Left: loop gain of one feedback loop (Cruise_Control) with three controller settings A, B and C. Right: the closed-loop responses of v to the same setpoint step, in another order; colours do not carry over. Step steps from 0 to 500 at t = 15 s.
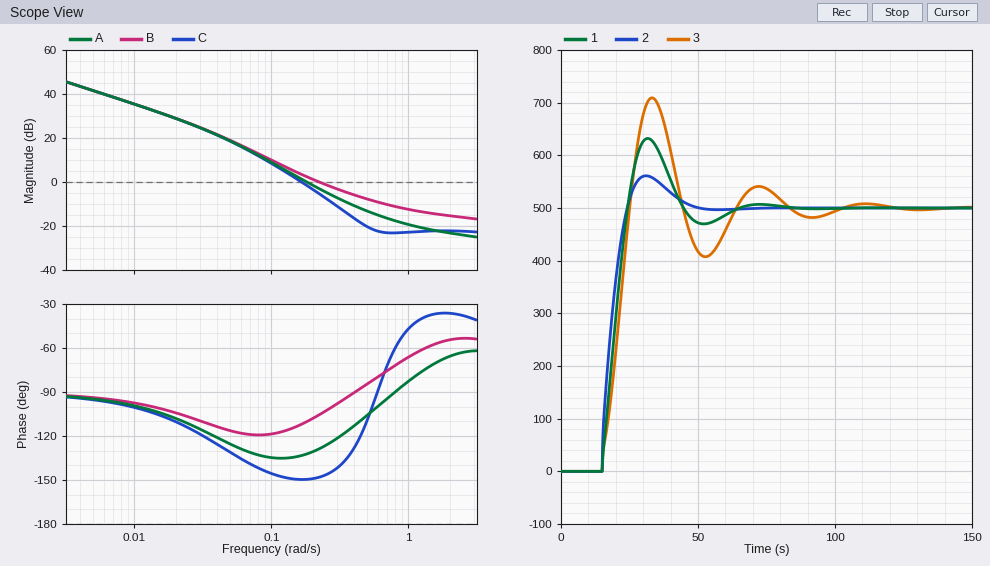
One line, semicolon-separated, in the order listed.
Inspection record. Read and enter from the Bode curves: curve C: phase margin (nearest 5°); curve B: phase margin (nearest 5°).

30°; 75°
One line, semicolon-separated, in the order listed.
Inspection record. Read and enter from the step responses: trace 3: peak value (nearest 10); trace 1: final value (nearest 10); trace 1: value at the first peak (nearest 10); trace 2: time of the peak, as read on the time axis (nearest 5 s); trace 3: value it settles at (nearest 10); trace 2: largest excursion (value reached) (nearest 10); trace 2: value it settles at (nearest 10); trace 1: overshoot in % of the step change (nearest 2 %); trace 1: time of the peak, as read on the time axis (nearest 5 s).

710; 500; 630; 30 s; 500; 560; 500; 26 %; 30 s
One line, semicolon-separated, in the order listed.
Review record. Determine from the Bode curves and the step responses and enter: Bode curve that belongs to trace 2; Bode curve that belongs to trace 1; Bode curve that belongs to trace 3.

B; A; C
